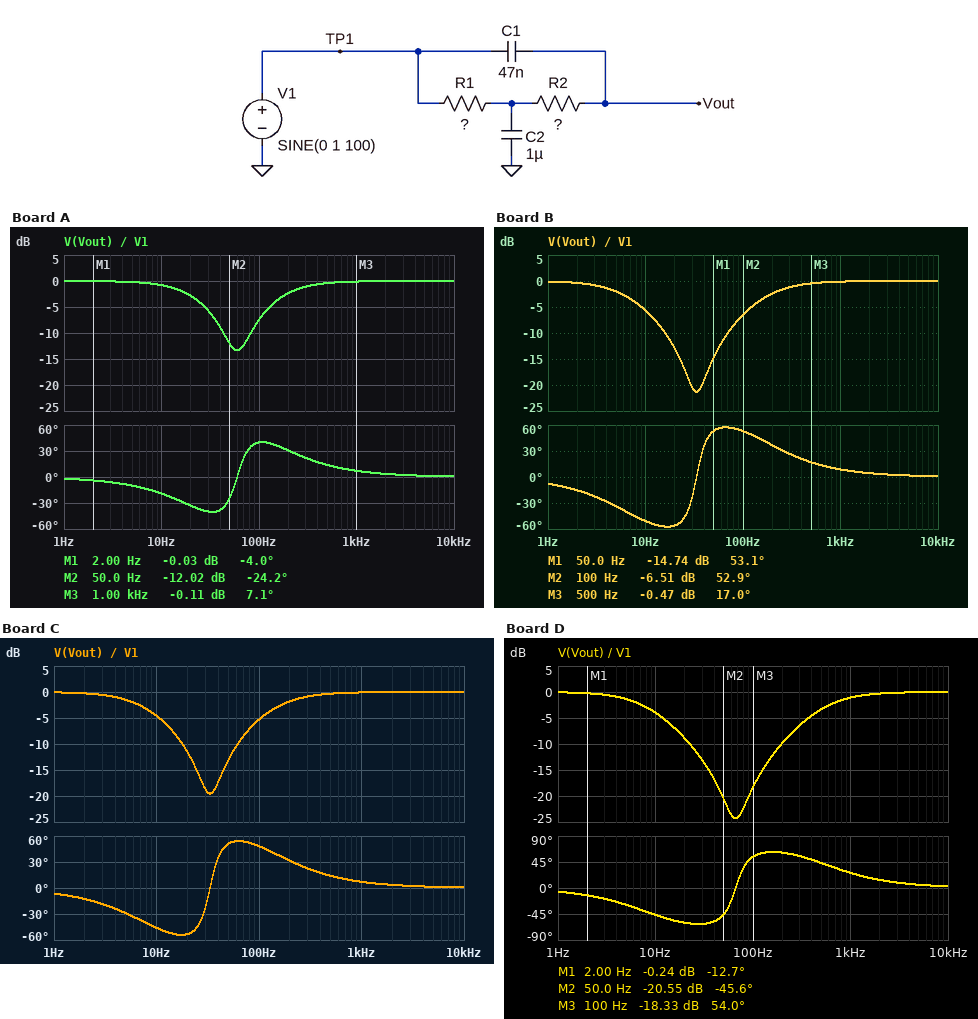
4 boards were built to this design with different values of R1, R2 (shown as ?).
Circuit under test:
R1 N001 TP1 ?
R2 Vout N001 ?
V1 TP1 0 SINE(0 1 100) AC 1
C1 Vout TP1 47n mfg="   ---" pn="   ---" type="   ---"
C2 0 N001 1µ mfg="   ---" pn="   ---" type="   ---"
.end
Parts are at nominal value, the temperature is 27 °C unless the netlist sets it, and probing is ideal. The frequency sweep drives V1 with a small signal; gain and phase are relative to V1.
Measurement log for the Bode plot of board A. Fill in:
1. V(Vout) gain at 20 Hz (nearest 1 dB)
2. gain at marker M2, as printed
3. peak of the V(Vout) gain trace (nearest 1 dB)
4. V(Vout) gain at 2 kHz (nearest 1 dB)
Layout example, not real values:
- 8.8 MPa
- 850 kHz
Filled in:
- -3 dB
- -12.02 dB
- 0 dB
- 0 dB
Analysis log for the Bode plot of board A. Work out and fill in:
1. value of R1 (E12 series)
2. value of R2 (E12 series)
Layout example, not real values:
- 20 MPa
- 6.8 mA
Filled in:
- 5.6 kΩ
- 27 kΩ
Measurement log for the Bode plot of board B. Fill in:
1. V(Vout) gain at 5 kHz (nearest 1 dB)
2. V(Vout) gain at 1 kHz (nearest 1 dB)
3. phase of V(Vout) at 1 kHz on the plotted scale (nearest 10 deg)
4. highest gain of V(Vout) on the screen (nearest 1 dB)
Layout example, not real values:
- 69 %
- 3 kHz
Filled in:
- 0 dB
- 0 dB
- 10 deg
- 0 dB
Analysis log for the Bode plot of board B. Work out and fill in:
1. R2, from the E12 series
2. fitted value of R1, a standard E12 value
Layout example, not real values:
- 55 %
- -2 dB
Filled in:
- 22 kΩ
- 22 kΩ
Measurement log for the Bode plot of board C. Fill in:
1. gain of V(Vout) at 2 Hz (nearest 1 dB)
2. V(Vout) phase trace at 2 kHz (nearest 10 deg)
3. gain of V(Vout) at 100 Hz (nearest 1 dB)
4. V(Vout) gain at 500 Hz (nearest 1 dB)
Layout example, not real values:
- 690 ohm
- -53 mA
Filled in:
- 0 dB
- 0 deg
- -5 dB
- 0 dB
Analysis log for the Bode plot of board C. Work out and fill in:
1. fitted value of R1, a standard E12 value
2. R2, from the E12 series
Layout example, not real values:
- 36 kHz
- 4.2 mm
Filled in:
- 18 kΩ
- 27 kΩ
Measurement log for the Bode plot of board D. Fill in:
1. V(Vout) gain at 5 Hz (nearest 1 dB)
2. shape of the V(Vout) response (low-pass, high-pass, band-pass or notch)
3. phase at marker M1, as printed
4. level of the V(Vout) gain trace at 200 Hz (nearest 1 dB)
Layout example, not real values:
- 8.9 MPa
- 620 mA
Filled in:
- -1 dB
- notch
- -12.7 deg
- -10 dB
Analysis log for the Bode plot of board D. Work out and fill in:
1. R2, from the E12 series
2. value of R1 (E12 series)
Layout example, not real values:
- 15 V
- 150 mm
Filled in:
- 6.8 kΩ
- 18 kΩ
